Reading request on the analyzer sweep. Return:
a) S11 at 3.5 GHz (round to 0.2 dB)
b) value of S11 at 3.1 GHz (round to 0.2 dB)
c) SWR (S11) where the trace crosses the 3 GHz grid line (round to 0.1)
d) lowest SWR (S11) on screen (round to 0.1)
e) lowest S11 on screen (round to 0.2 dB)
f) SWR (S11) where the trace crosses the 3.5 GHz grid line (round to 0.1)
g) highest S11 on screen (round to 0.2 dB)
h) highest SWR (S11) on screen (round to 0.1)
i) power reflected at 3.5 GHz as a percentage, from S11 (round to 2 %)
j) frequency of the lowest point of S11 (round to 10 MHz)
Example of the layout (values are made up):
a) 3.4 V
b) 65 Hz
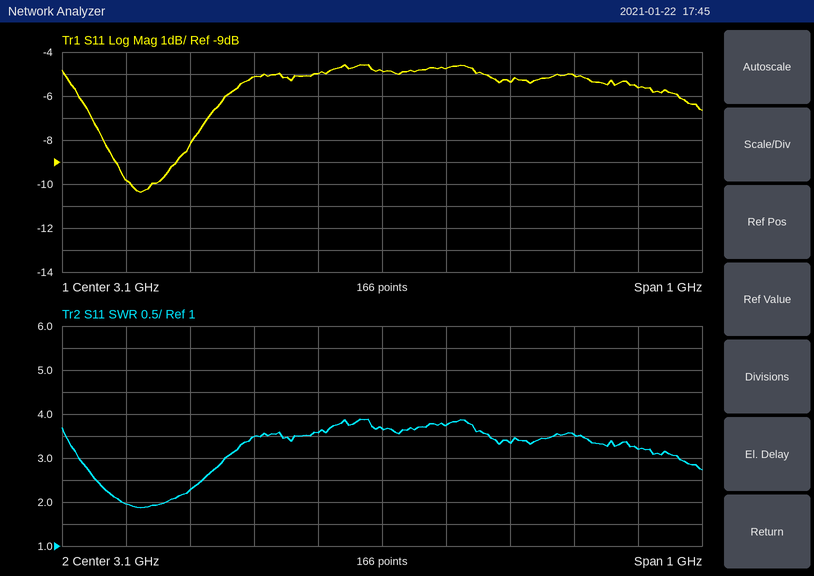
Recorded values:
a) -5.6 dB
b) -4.8 dB
c) 3.6
d) 1.9
e) -10.4 dB
f) 3.2
g) -4.6 dB
h) 3.9
i) 28 %
j) 2.72 GHz
